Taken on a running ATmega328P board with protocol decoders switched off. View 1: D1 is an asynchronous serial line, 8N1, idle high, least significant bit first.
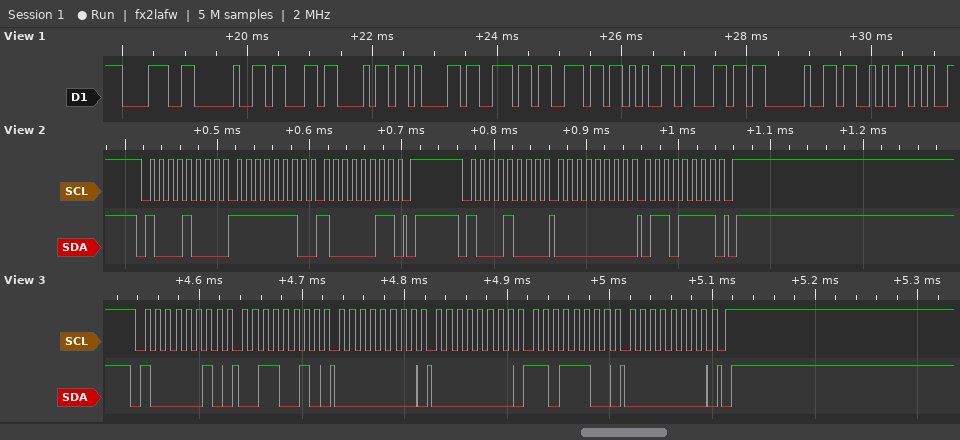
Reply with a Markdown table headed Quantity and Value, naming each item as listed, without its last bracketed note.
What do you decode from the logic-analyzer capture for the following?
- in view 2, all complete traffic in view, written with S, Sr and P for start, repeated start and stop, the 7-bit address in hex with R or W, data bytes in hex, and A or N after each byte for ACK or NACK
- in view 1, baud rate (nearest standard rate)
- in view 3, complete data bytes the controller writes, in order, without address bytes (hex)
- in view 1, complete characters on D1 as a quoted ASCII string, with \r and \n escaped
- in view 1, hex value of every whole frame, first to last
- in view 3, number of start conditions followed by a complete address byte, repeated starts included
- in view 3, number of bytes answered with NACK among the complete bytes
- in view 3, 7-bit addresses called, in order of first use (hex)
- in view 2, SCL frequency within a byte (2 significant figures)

| Quantity | Value |
|---|---|
| in view 2, all complete traffic in view, written with S, Sr and P for start, repeated start and stop, the 7-bit address in hex with R or W, data bytes in hex, and A or N after each byte for ACK or NACK | S 44W A FE A 83 A P S 44W A 00 A 6F A P |
| in view 1, baud rate | 9600 baud |
| in view 3, complete data bytes the controller writes, in order, without address bytes | 32 00 00 DC 00 |
| in view 1, complete characters on D1 as a quoted ASCII string, with \r and \n escaped | "8 channel S" |
| in view 1, hex value of every whole frame, first to last | 38 20 63 68 61 6E 6E 65 6C 20 53 |
| in view 3, number of start conditions followed by a complete address byte, repeated starts included | 1 |
| in view 3, number of bytes answered with NACK among the complete bytes | 0 |
| in view 3, 7-bit addresses called, in order of first use | 0x41 |
| in view 2, SCL frequency within a byte | 100 kHz |
